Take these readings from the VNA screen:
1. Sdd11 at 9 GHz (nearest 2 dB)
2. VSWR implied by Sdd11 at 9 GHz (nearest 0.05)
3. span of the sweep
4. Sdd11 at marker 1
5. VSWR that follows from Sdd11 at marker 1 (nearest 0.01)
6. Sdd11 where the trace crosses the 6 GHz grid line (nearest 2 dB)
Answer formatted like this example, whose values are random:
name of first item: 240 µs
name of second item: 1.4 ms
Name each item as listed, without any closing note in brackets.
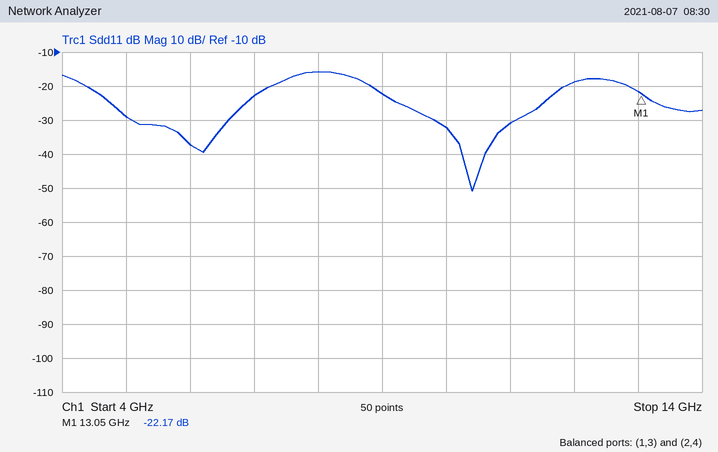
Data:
Sdd11 at 9 GHz: -22 dB
VSWR implied by Sdd11 at 9 GHz: 1.15
span of the sweep: 10 GHz
Sdd11 at marker 1: -22.17 dB
VSWR that follows from Sdd11 at marker 1: 1.17
Sdd11 where the trace crosses the 6 GHz grid line: -38 dB
